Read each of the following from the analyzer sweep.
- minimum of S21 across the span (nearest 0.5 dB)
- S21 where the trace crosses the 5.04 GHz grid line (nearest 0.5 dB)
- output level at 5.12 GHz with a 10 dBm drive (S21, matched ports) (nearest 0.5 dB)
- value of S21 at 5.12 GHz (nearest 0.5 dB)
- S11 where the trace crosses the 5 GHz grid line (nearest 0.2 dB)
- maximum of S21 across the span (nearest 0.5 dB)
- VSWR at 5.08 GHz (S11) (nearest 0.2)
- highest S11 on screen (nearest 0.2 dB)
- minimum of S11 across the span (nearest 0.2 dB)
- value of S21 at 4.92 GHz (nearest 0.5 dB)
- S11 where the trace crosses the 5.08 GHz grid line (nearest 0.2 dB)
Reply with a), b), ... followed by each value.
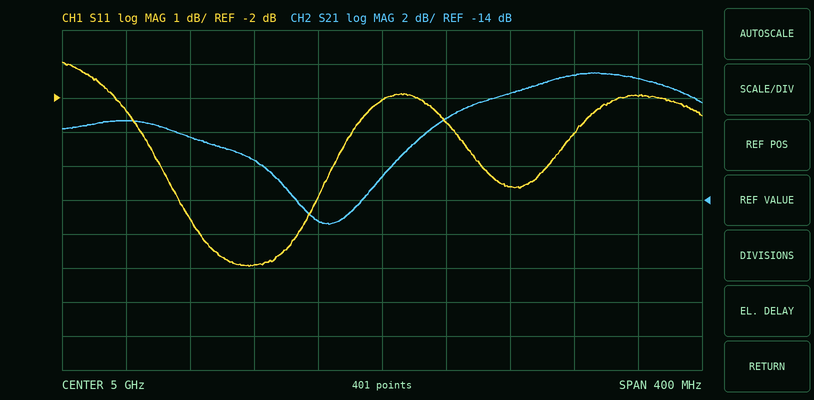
a) -15.5 dB
b) -9.0 dB
c) 3.5 dBm
d) -6.5 dB
e) -2.0 dB
f) -6.5 dB
g) 3.8
h) -1.0 dB
i) -7.0 dB
j) -11.5 dB
k) -4.6 dB
